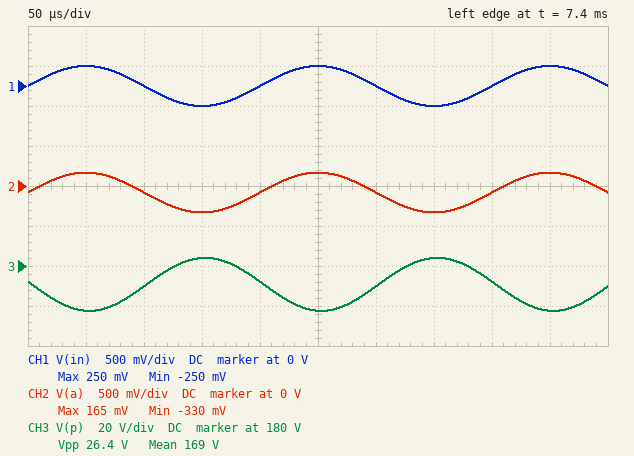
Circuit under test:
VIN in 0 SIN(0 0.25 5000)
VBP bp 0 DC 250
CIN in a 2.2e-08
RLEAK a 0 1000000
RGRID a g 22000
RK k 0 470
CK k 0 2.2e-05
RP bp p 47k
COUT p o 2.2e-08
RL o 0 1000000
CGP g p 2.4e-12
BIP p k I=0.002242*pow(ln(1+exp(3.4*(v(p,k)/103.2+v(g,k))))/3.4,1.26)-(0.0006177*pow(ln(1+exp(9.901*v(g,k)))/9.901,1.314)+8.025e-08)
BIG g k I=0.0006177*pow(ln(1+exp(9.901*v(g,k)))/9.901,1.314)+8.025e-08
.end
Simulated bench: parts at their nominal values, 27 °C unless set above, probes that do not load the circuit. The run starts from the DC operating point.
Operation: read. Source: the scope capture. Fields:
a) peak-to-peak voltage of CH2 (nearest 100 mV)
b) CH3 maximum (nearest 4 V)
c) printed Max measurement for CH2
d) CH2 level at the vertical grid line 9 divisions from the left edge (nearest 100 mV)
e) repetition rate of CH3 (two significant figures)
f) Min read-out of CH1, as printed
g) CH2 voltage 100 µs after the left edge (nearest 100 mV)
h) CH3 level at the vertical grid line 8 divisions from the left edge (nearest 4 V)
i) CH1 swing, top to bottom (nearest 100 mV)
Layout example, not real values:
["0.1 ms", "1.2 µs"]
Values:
["500 mV", "184 V", "165 mV", "200 mV", "5.0 kHz", "-250 mV", "-100 mV", "172 V", "500 mV"]
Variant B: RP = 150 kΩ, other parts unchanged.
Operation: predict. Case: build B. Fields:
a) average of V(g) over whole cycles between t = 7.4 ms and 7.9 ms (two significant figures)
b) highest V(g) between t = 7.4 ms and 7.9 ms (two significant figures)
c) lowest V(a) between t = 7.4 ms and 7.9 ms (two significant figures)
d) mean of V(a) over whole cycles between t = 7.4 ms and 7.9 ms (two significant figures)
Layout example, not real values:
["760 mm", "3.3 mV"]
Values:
["-130 mV", "110 mV", "-370 mV", "-120 mV"]
